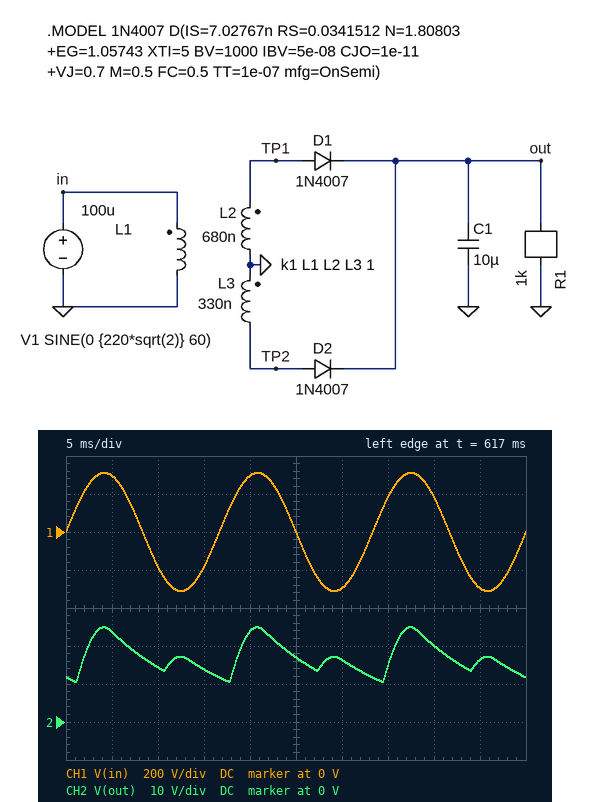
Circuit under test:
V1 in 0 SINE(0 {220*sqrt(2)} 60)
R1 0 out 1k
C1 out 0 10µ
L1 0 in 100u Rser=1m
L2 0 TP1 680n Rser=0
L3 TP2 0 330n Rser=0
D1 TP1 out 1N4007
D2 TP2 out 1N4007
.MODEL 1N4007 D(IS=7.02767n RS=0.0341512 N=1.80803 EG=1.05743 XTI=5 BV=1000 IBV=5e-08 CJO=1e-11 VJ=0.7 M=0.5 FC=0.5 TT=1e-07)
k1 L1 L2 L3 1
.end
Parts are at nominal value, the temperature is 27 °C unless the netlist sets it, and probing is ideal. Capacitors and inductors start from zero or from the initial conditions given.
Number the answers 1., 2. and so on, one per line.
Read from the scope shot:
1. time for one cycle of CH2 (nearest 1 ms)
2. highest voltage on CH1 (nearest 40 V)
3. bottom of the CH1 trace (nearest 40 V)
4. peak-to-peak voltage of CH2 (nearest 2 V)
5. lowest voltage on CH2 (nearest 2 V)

1. 17 ms
2. 320 V
3. -320 V
4. 14 V
5. 10 V
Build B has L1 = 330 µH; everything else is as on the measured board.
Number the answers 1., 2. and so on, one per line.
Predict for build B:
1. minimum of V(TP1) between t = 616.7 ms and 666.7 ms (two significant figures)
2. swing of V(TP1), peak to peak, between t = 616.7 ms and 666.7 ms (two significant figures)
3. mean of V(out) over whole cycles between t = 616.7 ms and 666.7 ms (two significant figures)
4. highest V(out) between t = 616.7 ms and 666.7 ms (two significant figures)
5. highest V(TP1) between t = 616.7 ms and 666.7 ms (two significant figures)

1. -14 V
2. 28 V
3. 9.2 V
4. 13 V
5. 14 V
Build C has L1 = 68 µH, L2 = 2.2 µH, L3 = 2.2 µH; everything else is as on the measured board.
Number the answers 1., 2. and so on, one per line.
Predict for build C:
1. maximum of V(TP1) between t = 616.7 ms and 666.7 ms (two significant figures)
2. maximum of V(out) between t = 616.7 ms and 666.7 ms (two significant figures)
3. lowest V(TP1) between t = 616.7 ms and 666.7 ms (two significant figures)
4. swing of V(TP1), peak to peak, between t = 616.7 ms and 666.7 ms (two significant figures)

1. 56 V
2. 55 V
3. -56 V
4. 110 V
